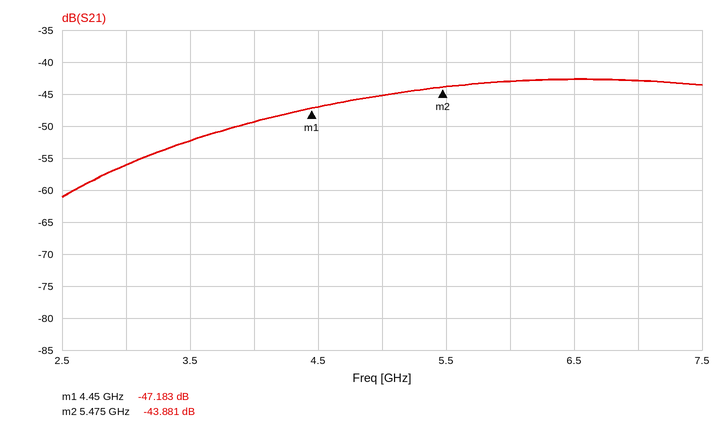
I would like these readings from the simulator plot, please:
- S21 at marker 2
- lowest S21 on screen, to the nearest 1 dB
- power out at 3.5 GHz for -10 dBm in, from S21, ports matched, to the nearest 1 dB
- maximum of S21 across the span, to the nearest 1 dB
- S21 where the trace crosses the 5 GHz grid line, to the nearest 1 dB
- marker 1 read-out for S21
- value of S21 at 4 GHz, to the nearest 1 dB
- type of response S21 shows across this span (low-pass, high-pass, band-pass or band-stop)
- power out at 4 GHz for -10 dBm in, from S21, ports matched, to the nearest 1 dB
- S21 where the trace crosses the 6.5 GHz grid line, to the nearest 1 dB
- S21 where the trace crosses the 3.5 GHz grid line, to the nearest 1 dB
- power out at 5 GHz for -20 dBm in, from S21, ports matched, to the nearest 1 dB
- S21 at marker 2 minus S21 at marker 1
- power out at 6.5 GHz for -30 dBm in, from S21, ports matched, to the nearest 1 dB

-43.881 dB
-61 dB
-62 dBm
-43 dB
-45 dB
-47.183 dB
-49 dB
high-pass
-59 dBm
-43 dB
-52 dB
-65 dBm
3.302 dB
-73 dBm
